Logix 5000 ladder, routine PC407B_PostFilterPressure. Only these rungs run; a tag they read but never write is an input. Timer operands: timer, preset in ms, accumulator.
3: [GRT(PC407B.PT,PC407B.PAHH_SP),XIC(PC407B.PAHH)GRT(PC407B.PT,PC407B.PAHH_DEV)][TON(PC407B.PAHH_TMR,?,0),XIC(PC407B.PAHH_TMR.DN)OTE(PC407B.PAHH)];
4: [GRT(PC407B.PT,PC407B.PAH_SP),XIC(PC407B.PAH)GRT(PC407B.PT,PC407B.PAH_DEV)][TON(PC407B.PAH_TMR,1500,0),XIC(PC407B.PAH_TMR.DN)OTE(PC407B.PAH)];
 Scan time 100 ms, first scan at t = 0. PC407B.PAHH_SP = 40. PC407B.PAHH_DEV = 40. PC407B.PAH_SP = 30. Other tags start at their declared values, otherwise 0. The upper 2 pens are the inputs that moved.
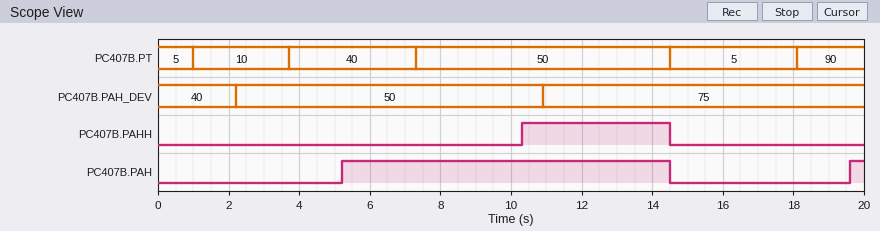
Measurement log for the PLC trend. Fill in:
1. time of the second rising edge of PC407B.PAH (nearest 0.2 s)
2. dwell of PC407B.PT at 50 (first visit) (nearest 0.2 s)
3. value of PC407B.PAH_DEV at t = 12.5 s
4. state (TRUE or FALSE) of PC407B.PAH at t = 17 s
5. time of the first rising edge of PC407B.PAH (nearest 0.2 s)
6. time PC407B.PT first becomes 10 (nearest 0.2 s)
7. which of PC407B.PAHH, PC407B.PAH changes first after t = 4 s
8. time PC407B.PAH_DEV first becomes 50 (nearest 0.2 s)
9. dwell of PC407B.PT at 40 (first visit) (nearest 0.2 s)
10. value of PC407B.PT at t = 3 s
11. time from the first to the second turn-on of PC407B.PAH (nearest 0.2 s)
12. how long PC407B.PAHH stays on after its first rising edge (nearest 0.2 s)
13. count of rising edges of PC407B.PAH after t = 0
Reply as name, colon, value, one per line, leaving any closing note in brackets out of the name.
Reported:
time of the second rising edge of PC407B.PAH: 19.6 s
dwell of PC407B.PT at 50 (first visit): 7.2 s
value of PC407B.PAH_DEV at t = 12.5 s: 75
state (TRUE or FALSE) of PC407B.PAH at t = 17 s: FALSE
time of the first rising edge of PC407B.PAH: 5.2 s
time PC407B.PT first becomes 10: 1.0 s
which of PC407B.PAHH, PC407B.PAH changes first after t = 4 s: PC407B.PAH
time PC407B.PAH_DEV first becomes 50: 2.2 s
dwell of PC407B.PT at 40 (first visit): 3.6 s
value of PC407B.PT at t = 3 s: 10
time from the first to the second turn-on of PC407B.PAH: 14.4 s
how long PC407B.PAHH stays on after its first rising edge: 4.2 s
count of rising edges of PC407B.PAH after t = 0: 2
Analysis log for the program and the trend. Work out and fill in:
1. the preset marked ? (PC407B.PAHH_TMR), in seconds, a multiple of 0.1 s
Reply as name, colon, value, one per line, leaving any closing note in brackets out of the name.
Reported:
the preset marked ? (PC407B.PAHH_TMR), in seconds, a multiple of 0.1 s: 3.0 s
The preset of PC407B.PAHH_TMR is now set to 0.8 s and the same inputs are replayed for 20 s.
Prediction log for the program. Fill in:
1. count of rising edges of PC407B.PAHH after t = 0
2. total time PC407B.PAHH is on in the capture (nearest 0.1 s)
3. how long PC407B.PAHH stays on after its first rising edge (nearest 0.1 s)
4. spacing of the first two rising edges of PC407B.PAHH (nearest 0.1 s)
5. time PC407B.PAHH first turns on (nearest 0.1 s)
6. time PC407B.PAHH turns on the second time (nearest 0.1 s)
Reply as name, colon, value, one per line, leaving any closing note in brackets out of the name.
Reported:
count of rising edges of PC407B.PAHH after t = 0: 2
total time PC407B.PAHH is on in the capture: 7.5 s
how long PC407B.PAHH stays on after its first rising edge: 6.4 s
spacing of the first two rising edges of PC407B.PAHH: 10.8 s
time PC407B.PAHH first turns on: 8.1 s
time PC407B.PAHH turns on the second time: 18.9 s
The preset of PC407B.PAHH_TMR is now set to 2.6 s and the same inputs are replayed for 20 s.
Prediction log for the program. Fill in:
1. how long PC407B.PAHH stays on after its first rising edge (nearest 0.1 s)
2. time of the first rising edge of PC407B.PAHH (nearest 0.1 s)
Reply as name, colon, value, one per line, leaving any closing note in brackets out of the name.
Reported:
how long PC407B.PAHH stays on after its first rising edge: 4.6 s
time of the first rising edge of PC407B.PAHH: 9.9 s
